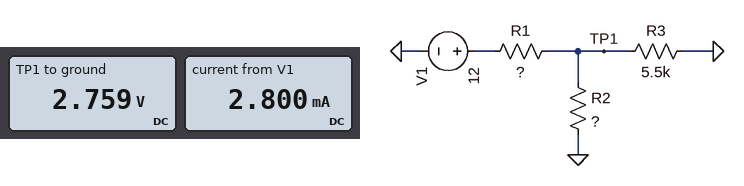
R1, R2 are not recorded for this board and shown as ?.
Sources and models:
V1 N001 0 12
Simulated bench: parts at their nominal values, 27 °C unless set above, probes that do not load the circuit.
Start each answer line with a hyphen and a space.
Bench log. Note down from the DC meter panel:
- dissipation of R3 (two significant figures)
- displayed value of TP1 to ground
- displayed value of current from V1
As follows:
- 1.4 mW
- 2.759 V
- 2.800 mA
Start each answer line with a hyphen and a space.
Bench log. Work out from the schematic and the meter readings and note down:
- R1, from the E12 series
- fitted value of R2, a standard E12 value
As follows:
- 3.3 kΩ
- 1.2 kΩ
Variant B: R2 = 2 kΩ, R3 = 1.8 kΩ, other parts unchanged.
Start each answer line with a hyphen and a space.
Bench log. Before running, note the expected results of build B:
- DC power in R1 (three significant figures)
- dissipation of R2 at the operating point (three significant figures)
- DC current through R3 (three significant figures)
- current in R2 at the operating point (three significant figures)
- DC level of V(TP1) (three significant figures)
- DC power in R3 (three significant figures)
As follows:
- 26.3 mW
- 3.58 mW
- 1.49 mA
- 1.34 mA
- 2.68 V
- 3.98 mW
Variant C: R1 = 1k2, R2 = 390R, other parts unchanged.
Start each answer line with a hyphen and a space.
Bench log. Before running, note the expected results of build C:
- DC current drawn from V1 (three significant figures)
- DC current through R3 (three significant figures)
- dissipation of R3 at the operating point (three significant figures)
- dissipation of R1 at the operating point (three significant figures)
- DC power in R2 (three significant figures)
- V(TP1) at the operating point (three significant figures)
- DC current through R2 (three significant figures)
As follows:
- 7.67 mA
- 508 µA
- 1.42 mW
- 70.6 mW
- 20.0 mW
- 2.79 V
- 7.16 mA
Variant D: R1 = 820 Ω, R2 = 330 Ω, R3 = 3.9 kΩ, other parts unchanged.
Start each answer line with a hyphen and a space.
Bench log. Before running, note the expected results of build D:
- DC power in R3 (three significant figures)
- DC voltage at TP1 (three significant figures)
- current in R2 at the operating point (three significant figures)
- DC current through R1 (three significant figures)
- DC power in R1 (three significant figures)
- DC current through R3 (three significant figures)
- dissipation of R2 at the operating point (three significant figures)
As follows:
- 2.70 mW
- 3.25 V
- 9.84 mA
- 10.7 mA
- 93.4 mW
- 833 µA
- 32.0 mW
